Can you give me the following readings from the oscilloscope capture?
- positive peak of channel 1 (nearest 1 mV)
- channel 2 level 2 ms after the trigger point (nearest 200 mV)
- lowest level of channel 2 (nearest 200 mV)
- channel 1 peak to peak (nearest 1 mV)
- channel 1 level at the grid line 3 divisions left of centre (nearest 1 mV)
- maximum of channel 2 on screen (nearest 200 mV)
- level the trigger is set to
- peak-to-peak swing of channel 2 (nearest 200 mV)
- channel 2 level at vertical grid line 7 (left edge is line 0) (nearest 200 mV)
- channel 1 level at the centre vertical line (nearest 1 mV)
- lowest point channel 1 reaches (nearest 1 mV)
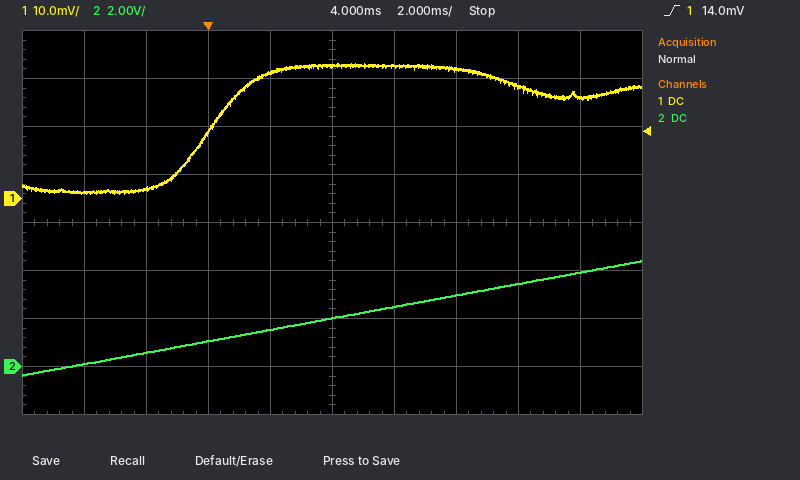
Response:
28 mV
1.6 V
-400 mV
27 mV
2 mV
4.4 V
14.0 mV
4.8 V
3.0 V
28 mV
1 mV
